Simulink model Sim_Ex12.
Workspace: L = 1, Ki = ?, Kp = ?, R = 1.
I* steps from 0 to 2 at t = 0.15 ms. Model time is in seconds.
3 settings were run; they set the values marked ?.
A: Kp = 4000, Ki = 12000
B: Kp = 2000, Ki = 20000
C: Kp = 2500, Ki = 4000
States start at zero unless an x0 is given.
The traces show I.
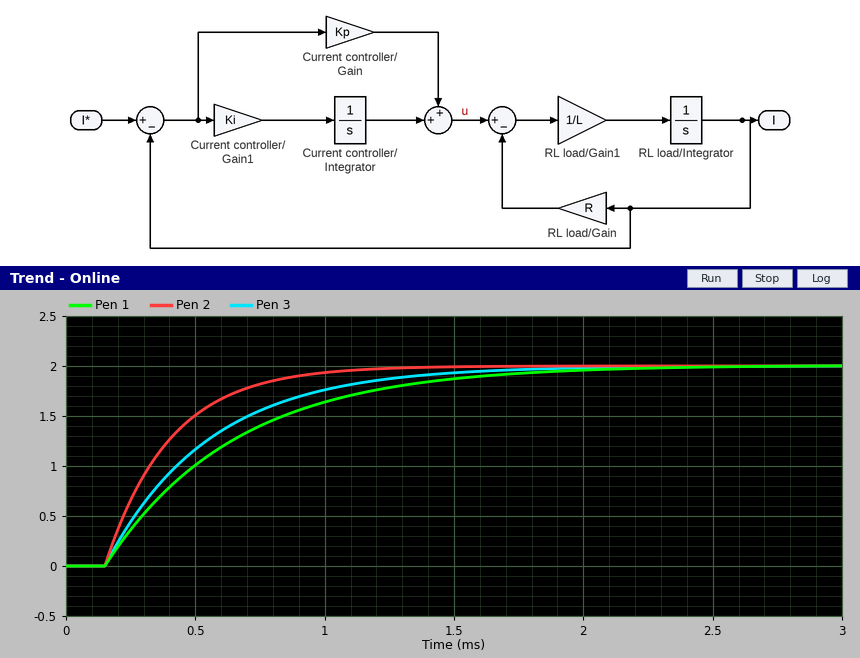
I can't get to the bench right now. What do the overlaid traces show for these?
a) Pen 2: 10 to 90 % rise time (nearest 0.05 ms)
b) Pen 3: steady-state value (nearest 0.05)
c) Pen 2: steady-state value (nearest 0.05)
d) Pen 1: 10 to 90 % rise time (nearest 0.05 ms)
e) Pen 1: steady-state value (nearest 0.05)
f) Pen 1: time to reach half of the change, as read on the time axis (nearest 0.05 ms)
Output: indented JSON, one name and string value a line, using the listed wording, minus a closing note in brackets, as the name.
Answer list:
{
  "Pen 2: 10 to 90 % rise time": "0.55 ms",
  "Pen 3: steady-state value": "2.00",
  "Pen 2: steady-state value": "2.00",
  "Pen 1: 10 to 90 % rise time": "1.10 ms",
  "Pen 1: steady-state value": "2.00",
  "Pen 1: time to reach half of the change, as read on the time axis": "0.50 ms"
}
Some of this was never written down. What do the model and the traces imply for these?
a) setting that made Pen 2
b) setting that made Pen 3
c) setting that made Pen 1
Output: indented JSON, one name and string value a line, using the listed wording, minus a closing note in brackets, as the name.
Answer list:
{
  "setting that made Pen 2": "A",
  "setting that made Pen 3": "C",
  "setting that made Pen 1": "B"
}
